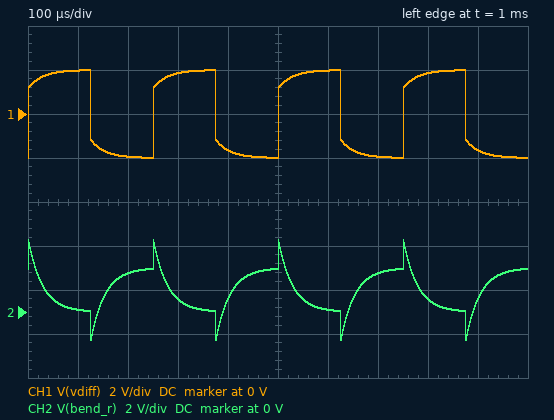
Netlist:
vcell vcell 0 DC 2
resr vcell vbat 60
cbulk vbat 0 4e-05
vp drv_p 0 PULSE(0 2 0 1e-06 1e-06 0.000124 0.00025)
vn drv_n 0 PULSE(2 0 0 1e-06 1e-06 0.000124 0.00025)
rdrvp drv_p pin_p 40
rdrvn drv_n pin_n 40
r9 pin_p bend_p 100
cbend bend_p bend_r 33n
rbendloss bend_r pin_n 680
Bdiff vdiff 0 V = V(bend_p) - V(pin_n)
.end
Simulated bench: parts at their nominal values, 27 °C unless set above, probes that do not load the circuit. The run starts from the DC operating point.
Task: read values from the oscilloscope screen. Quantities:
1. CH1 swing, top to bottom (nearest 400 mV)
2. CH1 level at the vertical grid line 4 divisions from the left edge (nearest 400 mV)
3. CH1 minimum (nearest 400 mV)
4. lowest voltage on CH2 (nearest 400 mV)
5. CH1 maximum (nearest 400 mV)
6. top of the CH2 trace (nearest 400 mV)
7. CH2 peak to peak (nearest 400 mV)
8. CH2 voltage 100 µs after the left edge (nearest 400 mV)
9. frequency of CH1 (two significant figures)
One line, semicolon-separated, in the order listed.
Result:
4.0 V; -1.6 V; -2.0 V; -1.2 V; 2.0 V; 3.2 V; 4.4 V; 0 V; 4.0 kHz
